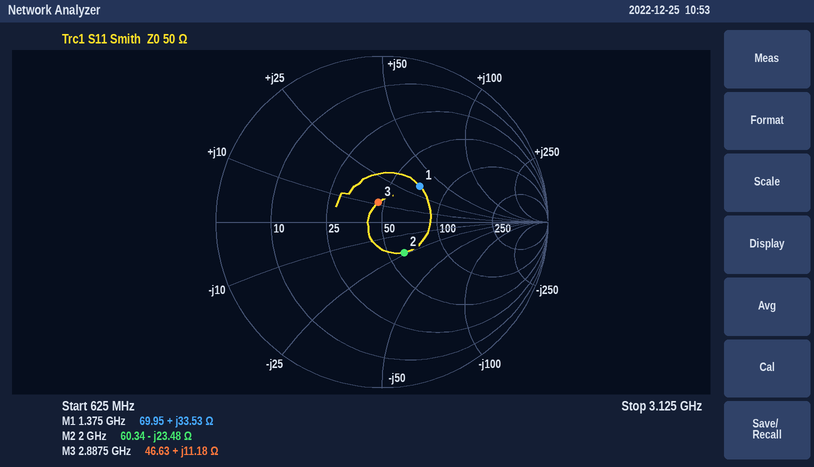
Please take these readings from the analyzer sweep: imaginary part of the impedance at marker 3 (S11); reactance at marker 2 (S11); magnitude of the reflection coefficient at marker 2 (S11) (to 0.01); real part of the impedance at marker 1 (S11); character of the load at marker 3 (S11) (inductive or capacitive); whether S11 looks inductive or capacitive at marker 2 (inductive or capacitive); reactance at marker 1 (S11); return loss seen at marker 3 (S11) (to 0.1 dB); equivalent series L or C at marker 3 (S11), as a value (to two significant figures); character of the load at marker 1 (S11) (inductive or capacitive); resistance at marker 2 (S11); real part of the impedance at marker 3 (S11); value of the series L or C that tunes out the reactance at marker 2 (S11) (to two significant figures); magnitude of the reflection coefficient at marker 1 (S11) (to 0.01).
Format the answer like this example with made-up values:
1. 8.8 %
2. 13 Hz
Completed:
1. +11.18 Ω
2. -23.48 Ω
3. 0.23
4. 69.95 Ω
5. inductive
6. capacitive
7. +33.53 Ω
8. 18.4 dB
9. 620 pH
10. inductive
11. 60.34 Ω
12. 46.63 Ω
13. 1.9 nH
14. 0.31
